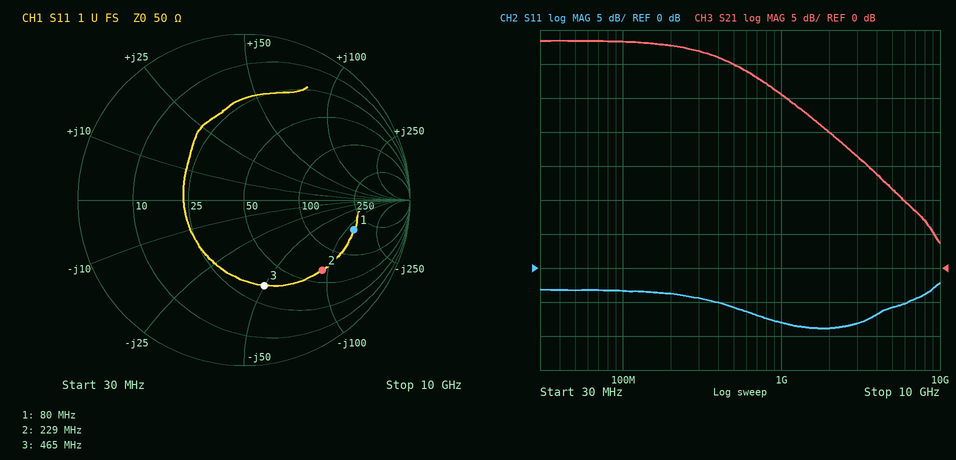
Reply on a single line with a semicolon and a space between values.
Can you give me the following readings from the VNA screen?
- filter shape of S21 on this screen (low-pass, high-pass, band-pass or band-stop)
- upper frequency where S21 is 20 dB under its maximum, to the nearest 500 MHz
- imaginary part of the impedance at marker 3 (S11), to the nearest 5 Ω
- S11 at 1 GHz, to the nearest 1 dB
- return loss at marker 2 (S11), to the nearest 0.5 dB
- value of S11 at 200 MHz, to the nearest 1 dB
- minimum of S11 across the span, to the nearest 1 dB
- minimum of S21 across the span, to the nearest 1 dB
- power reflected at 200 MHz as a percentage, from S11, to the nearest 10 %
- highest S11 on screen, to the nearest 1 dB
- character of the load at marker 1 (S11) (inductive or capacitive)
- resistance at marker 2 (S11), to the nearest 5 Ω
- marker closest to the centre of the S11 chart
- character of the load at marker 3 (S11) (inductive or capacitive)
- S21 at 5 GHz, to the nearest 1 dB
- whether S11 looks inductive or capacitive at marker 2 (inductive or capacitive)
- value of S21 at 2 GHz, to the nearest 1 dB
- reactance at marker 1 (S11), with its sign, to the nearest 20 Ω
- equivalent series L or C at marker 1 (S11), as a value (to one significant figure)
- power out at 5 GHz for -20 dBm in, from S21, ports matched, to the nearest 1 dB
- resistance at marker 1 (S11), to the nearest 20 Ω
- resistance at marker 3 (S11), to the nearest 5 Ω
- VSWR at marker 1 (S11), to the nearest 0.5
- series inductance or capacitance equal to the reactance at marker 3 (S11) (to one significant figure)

low-pass; 4.0 GHz; -50 Ω; -8 dB; 4.0 dB; -4 dB; -9 dB; 4 dB; 40 %; -2 dB; capacitive; 65 Ω; marker 3; capacitive; 12 dB; capacitive; 20 dB; -120 Ω; 20 pF; -8 dBm; 180 Ω; 35 Ω; 5.5; 7 pF
